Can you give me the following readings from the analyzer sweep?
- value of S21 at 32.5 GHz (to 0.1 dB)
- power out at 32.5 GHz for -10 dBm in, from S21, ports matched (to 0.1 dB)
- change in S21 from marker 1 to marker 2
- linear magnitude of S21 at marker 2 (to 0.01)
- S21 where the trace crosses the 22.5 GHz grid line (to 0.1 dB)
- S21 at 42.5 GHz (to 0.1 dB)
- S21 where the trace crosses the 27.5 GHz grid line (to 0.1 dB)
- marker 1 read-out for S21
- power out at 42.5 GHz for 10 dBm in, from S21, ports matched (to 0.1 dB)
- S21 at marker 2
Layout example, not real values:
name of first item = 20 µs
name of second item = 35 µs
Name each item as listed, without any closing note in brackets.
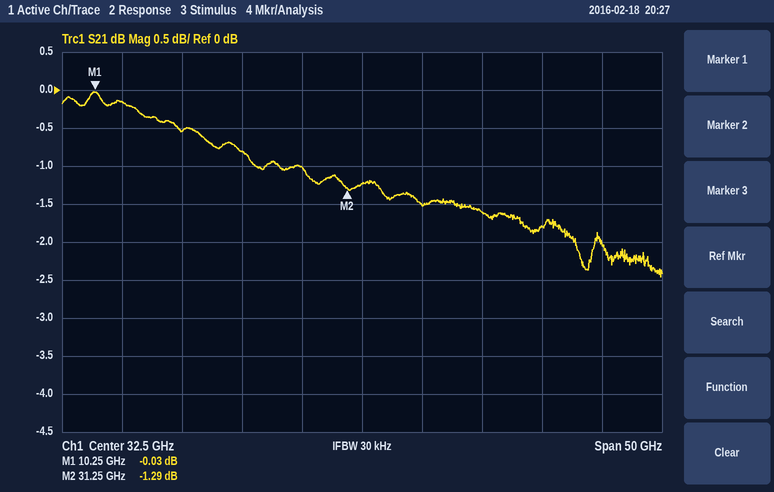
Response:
value of S21 at 32.5 GHz = -1.2 dB
power out at 32.5 GHz for -10 dBm in, from S21, ports matched = -11.2 dBm
change in S21 from marker 1 to marker 2 = -1.26 dB
linear magnitude of S21 at marker 2 = 0.86
S21 where the trace crosses the 22.5 GHz grid line = -0.8 dB
S21 at 42.5 GHz = -1.6 dB
S21 where the trace crosses the 27.5 GHz grid line = -1.0 dB
marker 1 read-out for S21 = -0.03 dB
power out at 42.5 GHz for 10 dBm in, from S21, ports matched = 8.4 dBm
S21 at marker 2 = -1.29 dB
